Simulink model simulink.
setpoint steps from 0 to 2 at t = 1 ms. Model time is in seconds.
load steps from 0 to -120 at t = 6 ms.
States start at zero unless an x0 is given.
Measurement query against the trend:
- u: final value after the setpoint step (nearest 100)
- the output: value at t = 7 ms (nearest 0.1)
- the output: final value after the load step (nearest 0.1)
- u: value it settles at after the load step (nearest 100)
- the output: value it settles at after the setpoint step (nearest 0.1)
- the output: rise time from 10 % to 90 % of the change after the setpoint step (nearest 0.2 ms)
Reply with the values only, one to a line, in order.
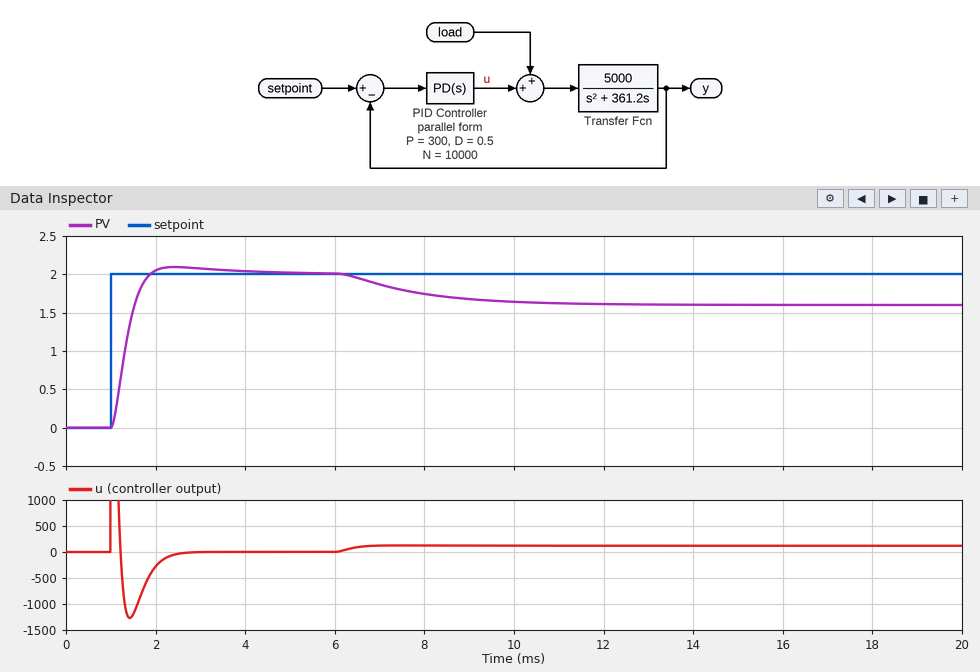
0
1.9
1.6
100
2.0
0.6 ms
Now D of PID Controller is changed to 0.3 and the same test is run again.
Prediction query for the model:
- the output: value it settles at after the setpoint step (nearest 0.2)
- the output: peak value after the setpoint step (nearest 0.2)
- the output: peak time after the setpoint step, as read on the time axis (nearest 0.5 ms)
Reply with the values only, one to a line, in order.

2.0
2.2
3.0 ms
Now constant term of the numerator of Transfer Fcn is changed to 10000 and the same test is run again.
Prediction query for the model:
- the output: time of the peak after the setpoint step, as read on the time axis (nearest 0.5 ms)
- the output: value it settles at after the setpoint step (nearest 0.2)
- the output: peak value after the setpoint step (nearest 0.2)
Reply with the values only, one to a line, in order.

1.5 ms
2.0
2.2
